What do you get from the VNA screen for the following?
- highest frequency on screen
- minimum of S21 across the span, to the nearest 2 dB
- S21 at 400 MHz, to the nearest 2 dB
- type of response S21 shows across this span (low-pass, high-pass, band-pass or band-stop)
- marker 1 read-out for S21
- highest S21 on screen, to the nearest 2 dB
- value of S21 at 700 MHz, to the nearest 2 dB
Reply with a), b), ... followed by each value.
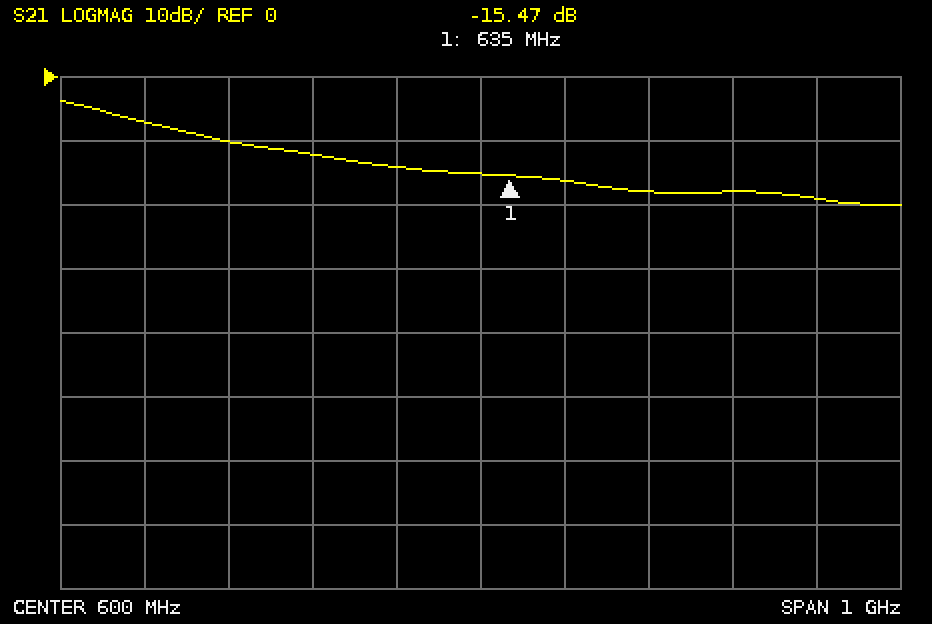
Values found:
a) 1.1 GHz
b) -20 dB
c) -12 dB
d) low-pass
e) -15.47 dB
f) -4 dB
g) -16 dB
